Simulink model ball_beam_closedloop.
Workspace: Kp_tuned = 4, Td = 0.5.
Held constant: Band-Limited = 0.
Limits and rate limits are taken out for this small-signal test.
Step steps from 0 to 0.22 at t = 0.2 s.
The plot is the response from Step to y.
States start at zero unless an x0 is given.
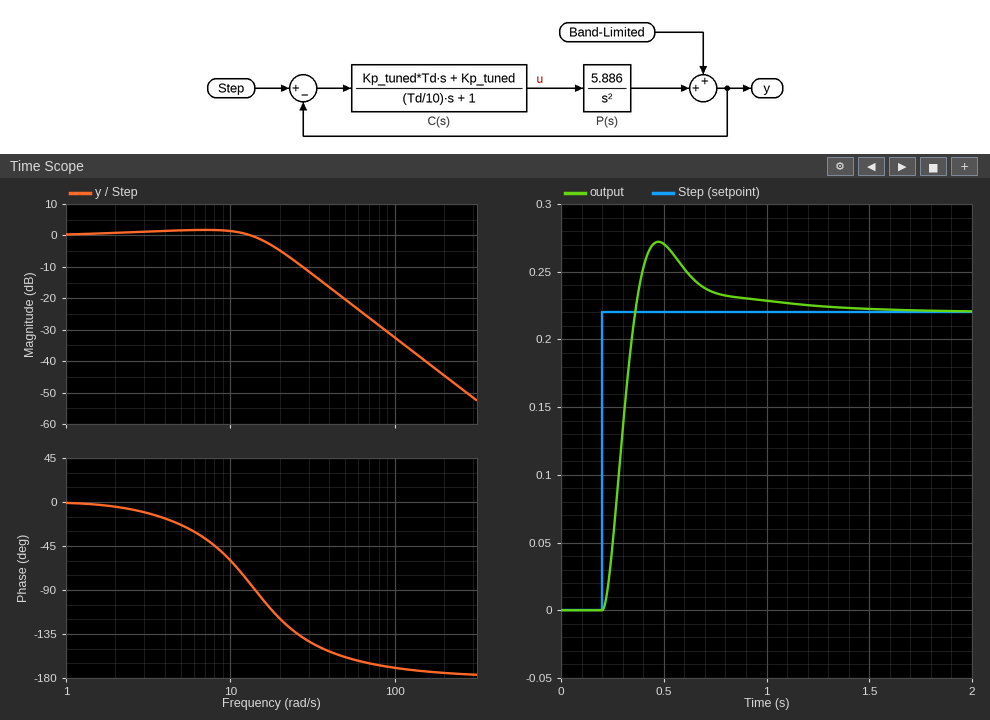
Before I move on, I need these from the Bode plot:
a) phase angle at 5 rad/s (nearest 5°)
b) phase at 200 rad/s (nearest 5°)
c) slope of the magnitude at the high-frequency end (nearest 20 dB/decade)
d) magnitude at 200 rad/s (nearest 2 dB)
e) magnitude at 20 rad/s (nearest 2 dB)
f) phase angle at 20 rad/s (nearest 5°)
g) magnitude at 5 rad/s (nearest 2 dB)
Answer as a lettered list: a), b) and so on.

a) -25°
b) -175°
c) -40 dB/decade
d) -44 dB
e) -4 dB
f) -120°
g) 2 dB
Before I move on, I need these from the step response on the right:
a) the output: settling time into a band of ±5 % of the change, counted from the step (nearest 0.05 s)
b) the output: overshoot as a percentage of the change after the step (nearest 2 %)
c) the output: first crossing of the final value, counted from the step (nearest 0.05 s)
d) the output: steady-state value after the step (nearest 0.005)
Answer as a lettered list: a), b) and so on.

a) 0.65 s
b) 24 %
c) 0.15 s
d) 0.220
